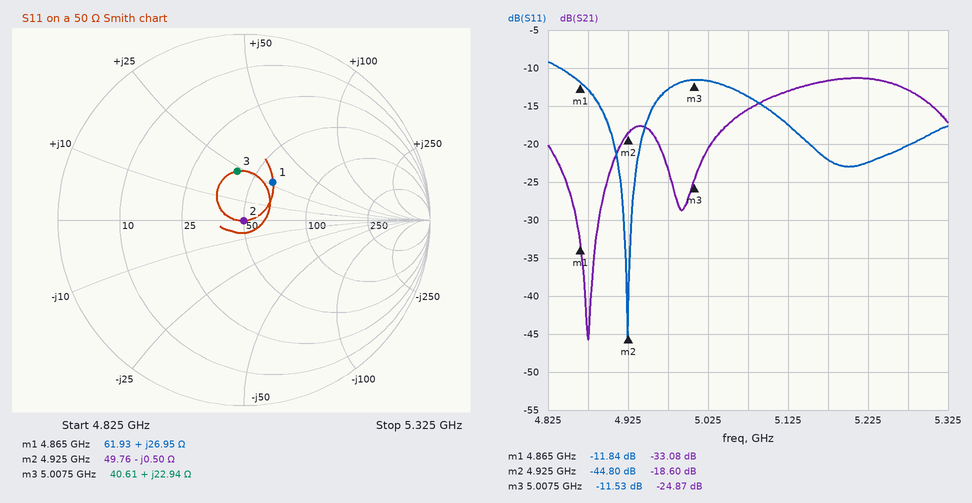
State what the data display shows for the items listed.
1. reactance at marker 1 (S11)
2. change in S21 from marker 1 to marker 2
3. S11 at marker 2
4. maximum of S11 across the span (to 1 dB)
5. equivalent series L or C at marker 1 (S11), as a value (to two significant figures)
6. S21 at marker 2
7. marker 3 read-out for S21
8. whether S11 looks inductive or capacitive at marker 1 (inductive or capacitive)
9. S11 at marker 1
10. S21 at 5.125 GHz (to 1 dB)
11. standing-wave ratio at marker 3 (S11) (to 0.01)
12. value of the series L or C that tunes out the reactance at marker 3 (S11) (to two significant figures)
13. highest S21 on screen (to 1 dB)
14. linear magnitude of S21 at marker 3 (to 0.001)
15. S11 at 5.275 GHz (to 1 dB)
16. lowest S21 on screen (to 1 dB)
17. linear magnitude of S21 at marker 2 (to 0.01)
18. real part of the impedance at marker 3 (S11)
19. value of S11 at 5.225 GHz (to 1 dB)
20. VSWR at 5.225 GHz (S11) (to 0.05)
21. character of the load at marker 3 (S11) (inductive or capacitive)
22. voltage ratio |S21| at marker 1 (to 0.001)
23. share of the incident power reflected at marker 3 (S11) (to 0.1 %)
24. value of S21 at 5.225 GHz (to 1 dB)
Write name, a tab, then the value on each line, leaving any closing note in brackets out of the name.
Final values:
reactance at marker 1	+26.95 Ω
change in S21 from marker 1 to marker 2	14.48 dB
S11 at marker 2	-44.80 dB
maximum of S11 across the span	-9 dB
equivalent series L or C at marker 1 (S11), as a value	880 pH
S21 at marker 2	-18.60 dB
marker 3 read-out for S21	-24.87 dB
whether S11 looks inductive or capacitive at marker 1	inductive
S11 at marker 1	-11.84 dB
S21 at 5.125 GHz	-13 dB
standing-wave ratio at marker 3 (S11)	1.72
value of the series L or C that tunes out the reactance at marker 3 (S11)	1.4 pF
highest S21 on screen	-11 dB
linear magnitude of S21 at marker 3	0.057
S11 at 5.275 GHz	-20 dB
lowest S21 on screen	-46 dB
linear magnitude of S21 at marker 2	0.12
real part of the impedance at marker 3	40.61 Ω
value of S11 at 5.225 GHz	-22 dB
VSWR at 5.225 GHz (S11)	1.15
character of the load at marker 3 (S11)	inductive
voltage ratio |S21| at marker 1	0.022
share of the incident power reflected at marker 3 (S11)	7.0 %
value of S21 at 5.225 GHz	-11 dB
